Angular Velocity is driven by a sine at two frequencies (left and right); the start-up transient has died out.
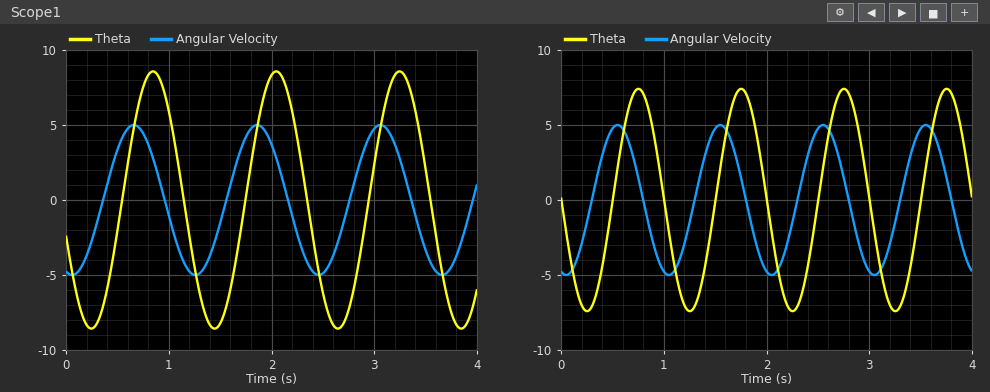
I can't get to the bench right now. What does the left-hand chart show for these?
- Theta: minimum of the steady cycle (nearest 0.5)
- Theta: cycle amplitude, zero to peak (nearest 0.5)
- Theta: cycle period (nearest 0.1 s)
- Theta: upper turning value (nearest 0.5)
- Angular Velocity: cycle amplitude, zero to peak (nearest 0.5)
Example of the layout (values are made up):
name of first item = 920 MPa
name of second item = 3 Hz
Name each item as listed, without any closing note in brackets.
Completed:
Theta: minimum of the steady cycle = -8.5
Theta: cycle amplitude, zero to peak = 8.5
Theta: cycle period = 1.2 s
Theta: upper turning value = 8.5
Angular Velocity: cycle amplitude, zero to peak = 5.0
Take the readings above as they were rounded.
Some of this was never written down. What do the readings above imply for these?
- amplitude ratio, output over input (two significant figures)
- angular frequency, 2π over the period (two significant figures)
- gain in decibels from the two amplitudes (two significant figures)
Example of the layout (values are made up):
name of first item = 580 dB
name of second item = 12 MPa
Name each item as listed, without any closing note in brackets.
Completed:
amplitude ratio, output over input = 1.7
angular frequency, 2π over the period = 5.2 rad/s
gain in decibels from the two amplitudes = 4.6 dB
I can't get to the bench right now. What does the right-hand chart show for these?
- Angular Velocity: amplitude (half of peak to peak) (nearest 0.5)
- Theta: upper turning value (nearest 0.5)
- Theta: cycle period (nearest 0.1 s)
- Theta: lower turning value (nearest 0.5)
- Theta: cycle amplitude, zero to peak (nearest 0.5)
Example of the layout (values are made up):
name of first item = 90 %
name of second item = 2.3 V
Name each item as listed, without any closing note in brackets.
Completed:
Angular Velocity: amplitude (half of peak to peak) = 5.0
Theta: upper turning value = 7.5
Theta: cycle period = 1.0 s
Theta: lower turning value = -7.5
Theta: cycle amplitude, zero to peak = 7.5
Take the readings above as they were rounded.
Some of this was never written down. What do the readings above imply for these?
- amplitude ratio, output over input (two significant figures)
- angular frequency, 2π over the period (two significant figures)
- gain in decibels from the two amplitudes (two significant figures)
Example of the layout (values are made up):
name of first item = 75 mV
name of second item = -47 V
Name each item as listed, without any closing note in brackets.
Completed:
amplitude ratio, output over input = 1.5
angular frequency, 2π over the period = 6.3 rad/s
gain in decibels from the two amplitudes = 3.5 dB
